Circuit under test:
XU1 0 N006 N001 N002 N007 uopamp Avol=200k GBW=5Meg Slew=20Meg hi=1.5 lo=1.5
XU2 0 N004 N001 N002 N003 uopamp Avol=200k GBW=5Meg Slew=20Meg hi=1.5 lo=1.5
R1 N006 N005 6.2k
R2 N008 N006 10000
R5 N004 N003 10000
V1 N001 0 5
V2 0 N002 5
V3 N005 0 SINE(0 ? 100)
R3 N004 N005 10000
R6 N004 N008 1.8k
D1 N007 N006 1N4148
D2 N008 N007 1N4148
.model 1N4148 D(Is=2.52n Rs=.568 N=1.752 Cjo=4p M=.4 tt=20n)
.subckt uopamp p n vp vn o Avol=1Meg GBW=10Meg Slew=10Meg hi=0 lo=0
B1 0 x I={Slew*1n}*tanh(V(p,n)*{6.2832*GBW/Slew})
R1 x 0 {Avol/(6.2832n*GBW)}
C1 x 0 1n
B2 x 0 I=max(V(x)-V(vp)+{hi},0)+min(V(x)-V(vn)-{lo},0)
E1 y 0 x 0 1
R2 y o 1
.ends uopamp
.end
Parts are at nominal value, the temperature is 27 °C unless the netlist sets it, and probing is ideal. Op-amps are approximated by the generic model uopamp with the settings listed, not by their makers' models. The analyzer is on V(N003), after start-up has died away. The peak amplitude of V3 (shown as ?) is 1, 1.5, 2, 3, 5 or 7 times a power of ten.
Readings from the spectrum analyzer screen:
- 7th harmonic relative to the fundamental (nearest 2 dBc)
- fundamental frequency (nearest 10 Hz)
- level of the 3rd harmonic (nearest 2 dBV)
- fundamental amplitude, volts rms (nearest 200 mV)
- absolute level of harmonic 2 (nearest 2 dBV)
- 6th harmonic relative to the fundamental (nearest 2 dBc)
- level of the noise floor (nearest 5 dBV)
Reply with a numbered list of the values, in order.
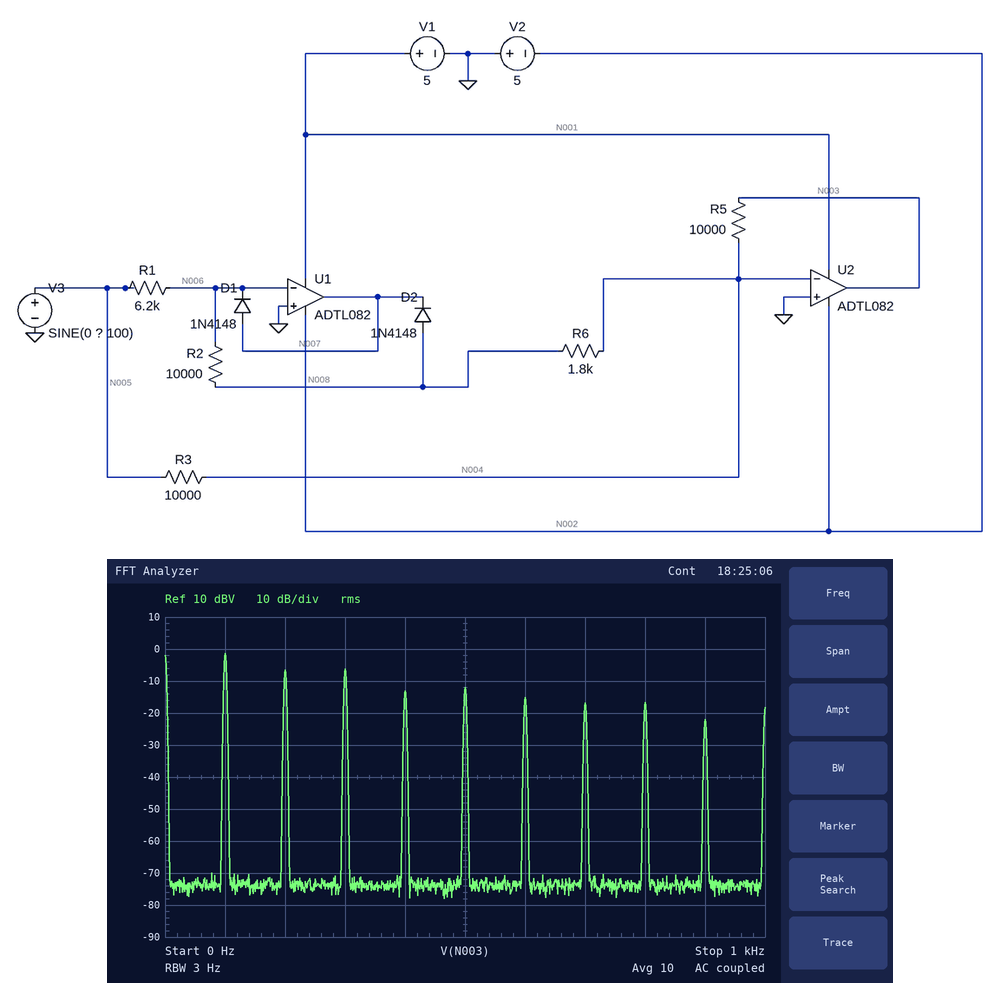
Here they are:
1. -16 dBc
2. 100 Hz
3. -6 dBV
4. 800 mV
5. -6 dBV
6. -14 dBc
7. -75 dBV
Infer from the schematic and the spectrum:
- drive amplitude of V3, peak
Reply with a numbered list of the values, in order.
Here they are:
1. 2 V
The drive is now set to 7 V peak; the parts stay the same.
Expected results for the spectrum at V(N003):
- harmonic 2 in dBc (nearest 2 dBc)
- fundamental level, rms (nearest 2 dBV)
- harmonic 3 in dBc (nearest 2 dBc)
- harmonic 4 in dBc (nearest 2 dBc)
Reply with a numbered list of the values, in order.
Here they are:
1. 16 dBc
2. -24 dBV
3. 8 dBc
4. 14 dBc
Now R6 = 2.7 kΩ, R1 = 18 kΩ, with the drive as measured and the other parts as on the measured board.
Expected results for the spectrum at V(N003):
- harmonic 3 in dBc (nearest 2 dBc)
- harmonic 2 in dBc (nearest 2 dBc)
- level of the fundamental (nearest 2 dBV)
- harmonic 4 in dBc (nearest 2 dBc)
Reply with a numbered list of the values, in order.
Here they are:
1. -60 dBc
2. 24 dBc
3. -28 dBV
4. 10 dBc
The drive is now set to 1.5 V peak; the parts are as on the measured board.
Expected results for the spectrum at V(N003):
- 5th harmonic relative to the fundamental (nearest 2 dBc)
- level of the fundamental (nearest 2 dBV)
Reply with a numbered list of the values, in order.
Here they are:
1. -14 dBc
2. 0 dBV
